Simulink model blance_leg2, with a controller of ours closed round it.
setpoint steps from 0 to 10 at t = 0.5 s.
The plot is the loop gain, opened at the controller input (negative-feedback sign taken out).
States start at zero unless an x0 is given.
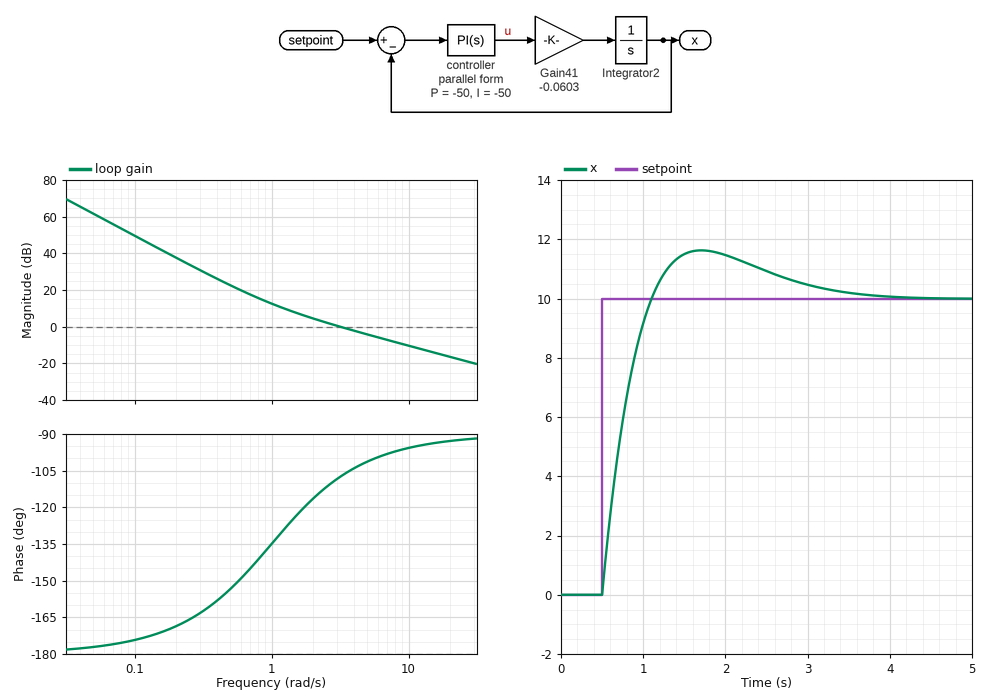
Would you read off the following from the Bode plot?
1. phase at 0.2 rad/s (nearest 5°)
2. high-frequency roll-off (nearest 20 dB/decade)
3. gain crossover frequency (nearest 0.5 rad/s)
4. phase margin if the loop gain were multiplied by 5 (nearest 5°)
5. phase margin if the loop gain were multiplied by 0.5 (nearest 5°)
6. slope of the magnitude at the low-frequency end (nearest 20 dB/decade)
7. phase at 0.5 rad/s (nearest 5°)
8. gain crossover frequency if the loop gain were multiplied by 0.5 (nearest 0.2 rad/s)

-170°
-20 dB/decade
3.0 rad/s
85°
60°
-40 dB/decade
-155°
1.8 rad/s
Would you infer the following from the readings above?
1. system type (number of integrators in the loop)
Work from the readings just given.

2
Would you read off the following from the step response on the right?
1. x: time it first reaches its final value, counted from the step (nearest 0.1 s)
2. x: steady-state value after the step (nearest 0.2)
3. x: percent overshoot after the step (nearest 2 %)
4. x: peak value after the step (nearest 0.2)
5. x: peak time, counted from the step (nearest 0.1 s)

0.6 s
10.0
16 %
11.6
1.2 s
